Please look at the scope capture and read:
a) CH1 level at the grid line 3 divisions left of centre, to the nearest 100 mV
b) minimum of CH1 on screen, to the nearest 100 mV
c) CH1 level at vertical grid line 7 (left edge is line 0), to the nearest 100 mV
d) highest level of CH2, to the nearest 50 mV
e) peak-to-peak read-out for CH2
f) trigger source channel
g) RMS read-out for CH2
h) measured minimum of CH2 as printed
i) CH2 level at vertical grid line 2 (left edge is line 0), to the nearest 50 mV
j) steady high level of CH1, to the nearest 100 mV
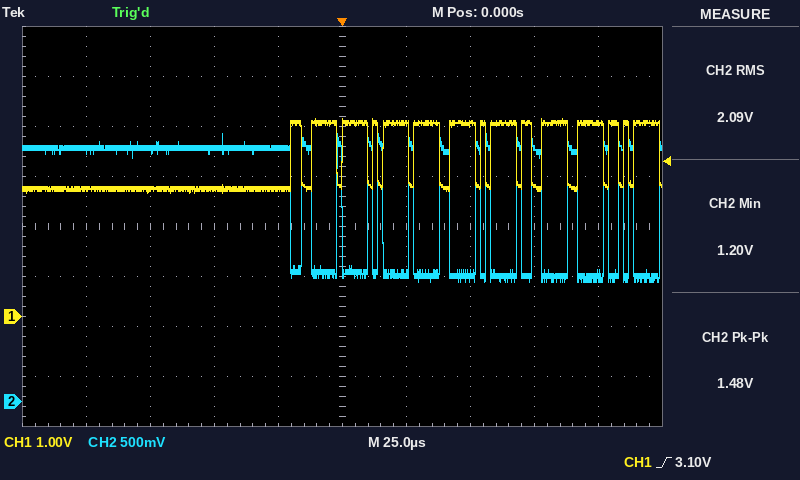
2.5 V
2.5 V
3.9 V
2.70 V
1.48 V
CH1
2.09 V
1.20 V
2.50 V
3.9 V
